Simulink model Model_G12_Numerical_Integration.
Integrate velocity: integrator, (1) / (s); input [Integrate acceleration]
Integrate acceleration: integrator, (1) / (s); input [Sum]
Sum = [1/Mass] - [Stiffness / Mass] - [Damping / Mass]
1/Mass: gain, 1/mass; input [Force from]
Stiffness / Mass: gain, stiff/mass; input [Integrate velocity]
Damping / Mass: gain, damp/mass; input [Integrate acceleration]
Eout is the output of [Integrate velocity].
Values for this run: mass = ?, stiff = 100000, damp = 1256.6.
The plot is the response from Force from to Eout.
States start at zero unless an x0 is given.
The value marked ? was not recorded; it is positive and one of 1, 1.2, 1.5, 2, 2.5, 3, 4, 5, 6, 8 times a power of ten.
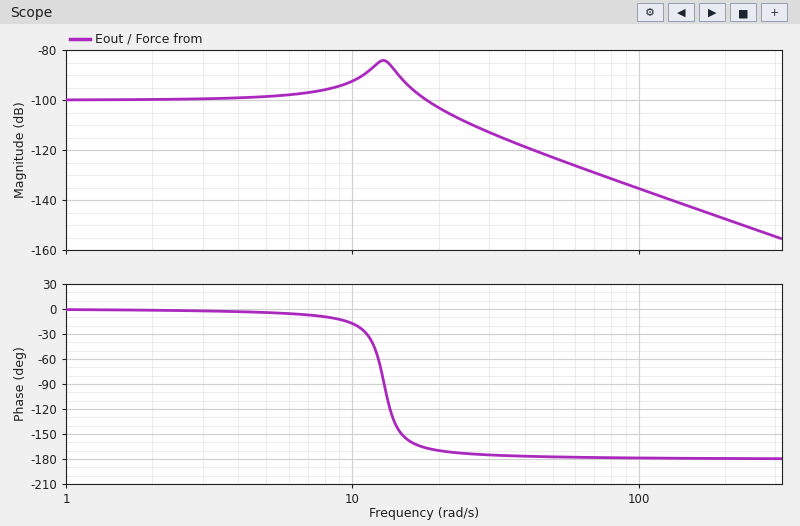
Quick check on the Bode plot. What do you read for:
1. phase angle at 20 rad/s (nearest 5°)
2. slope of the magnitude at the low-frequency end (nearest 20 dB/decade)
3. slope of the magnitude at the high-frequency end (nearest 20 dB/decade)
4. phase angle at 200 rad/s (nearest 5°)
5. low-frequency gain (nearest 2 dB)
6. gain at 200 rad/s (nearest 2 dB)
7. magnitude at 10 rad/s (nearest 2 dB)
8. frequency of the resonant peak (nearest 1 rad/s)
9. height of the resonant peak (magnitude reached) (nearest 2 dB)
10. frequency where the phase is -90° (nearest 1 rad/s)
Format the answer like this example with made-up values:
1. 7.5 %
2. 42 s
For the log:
1. -170°
2. 0 dB/decade
3. -40 dB/decade
4. -180°
5. -100 dB
6. -148 dB
7. -92 dB
8. 13 rad/s
9. -84 dB
10. 13 rad/s
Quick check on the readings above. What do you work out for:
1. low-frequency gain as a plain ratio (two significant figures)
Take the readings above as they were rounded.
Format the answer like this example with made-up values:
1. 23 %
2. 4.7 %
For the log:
1. 0.000010
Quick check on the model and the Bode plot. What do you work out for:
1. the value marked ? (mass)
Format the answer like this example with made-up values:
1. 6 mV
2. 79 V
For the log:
1. 600
